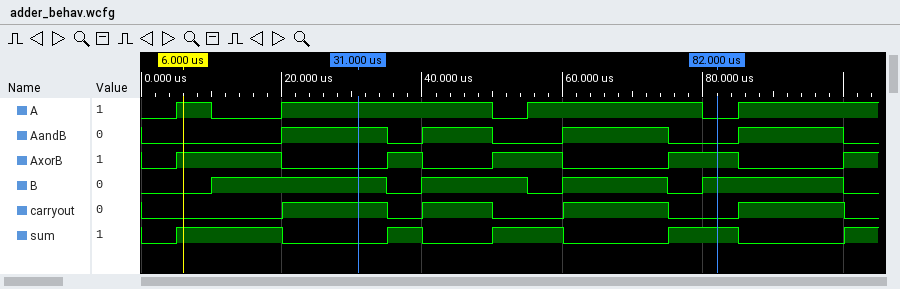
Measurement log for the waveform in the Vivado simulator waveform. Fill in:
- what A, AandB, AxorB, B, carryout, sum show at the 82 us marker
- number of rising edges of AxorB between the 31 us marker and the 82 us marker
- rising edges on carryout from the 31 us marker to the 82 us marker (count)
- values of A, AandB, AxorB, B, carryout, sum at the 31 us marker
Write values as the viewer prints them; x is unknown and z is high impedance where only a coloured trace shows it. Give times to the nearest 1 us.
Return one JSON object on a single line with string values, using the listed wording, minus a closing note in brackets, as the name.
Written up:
{"what A, AandB, AxorB, B, carryout, sum show at the 82 us marker": "A=0, AandB=0, AxorB=1, B=1, carryout=0, sum=1", "number of rising edges of AxorB between the 31 us marker and the 82 us marker": "3", "rising edges on carryout from the 31 us marker to the 82 us marker": "2", "values of A, AandB, AxorB, B, carryout, sum at the 31 us marker": "A=1, AandB=1, AxorB=0, B=1, carryout=1, sum=0"}
